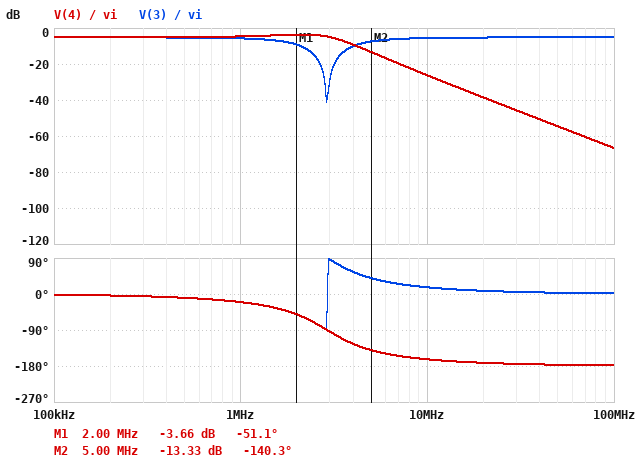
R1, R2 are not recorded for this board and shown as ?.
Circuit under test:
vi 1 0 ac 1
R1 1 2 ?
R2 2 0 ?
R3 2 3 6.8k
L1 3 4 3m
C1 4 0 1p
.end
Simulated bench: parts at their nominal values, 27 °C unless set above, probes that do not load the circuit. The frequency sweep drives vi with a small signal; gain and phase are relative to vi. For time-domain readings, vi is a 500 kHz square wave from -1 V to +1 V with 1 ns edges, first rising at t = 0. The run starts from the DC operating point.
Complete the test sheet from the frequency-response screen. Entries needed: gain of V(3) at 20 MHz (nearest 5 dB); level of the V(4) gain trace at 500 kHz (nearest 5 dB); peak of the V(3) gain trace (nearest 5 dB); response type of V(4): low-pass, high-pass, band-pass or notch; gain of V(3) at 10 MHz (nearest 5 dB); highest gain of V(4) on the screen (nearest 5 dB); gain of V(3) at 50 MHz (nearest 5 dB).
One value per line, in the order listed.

-5 dB
-5 dB
-5 dB
low-pass
-5 dB
-5 dB
-5 dB
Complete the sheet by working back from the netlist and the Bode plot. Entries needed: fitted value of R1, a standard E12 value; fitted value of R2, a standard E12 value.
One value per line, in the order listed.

82 kΩ
100 kΩ
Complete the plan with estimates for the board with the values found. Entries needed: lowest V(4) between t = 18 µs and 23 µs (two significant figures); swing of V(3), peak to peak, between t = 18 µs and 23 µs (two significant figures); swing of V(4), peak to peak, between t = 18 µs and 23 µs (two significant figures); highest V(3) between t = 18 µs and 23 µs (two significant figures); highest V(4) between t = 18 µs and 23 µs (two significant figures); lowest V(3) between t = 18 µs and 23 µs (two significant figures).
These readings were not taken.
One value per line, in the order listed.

-750 mV
1.3 V
1.5 V
660 mV
750 mV
-660 mV
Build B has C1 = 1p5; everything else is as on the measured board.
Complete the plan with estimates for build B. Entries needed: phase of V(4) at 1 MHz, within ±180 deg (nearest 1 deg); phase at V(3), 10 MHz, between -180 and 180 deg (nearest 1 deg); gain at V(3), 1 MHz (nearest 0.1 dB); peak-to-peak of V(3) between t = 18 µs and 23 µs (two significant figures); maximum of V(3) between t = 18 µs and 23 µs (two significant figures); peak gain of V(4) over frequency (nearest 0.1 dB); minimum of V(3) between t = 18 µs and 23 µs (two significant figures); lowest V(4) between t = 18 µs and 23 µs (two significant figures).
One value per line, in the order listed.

-31 deg
16 deg
-6.5 dB
1.2 V
620 mV
-4.7 dB
-620 mV
-670 mV
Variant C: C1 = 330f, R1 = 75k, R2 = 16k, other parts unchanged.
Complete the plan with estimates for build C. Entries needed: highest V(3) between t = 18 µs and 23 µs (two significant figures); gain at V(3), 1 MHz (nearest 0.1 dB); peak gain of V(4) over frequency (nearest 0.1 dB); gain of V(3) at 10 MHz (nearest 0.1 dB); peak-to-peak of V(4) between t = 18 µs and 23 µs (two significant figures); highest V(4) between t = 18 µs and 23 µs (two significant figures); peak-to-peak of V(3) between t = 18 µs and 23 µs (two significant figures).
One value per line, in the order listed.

220 mV
-15.1 dB
-1.5 dB
-15.2 dB
840 mV
420 mV
440 mV
